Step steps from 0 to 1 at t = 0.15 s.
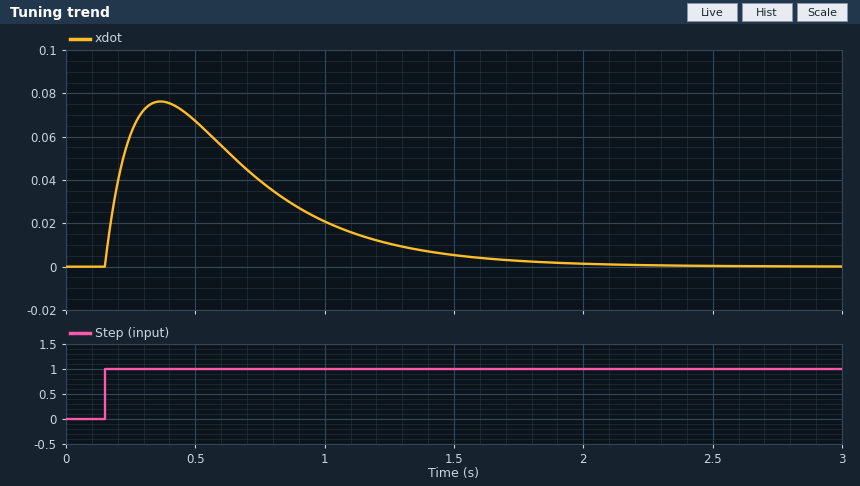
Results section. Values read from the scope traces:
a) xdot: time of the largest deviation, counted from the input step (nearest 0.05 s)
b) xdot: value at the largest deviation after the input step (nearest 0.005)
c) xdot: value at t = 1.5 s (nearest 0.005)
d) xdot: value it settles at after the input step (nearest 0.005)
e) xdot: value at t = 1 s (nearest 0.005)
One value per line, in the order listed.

0.20 s
0.075
0.005
0.000
0.020
